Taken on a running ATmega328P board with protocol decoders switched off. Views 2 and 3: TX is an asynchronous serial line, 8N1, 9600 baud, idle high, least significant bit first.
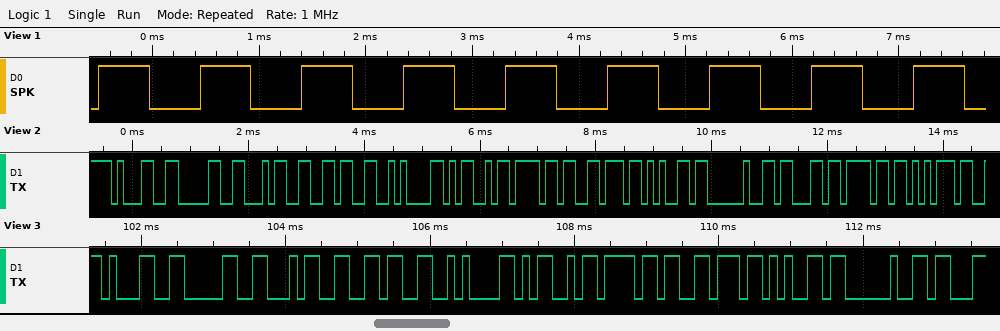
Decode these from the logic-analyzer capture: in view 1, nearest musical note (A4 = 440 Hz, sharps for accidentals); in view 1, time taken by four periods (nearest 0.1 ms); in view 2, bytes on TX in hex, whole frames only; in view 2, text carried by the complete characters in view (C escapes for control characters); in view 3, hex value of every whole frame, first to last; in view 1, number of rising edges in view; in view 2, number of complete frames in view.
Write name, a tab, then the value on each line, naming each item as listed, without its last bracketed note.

in view 1, nearest musical note	C6
in view 1, time taken by four periods	3.8 ms
in view 2, bytes on TX in hex, whole frames only	31 30 34 36 0A 4D 6F 76 65 20 63 6F 75
in view 2, text carried by the complete characters in view	"1046\nMove cou"
in view 3, hex value of every whole frame, first to last	31 30 34 36 0A 4D 6F 76 65 20
in view 1, number of rising edges in view	9
in view 2, number of complete frames in view	13
